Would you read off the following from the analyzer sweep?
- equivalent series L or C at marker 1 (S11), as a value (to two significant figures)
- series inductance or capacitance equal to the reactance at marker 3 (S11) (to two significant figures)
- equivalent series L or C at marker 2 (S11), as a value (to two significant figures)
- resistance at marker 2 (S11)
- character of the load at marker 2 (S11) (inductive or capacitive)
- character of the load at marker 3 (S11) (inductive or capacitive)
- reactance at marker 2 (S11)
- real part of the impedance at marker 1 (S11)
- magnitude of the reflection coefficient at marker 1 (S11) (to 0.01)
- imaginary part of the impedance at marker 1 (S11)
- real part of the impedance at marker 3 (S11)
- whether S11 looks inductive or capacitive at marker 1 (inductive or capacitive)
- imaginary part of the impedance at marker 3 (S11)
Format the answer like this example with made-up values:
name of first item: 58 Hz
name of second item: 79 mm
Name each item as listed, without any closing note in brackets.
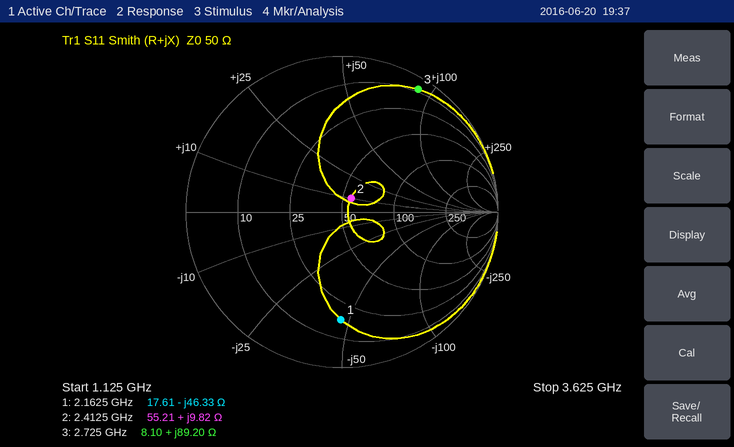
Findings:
equivalent series L or C at marker 1 (S11), as a value: 1.6 pF
series inductance or capacitance equal to the reactance at marker 3 (S11): 5.2 nH
equivalent series L or C at marker 2 (S11), as a value: 650 pH
resistance at marker 2: 55.21 Ω
character of the load at marker 2 (S11): inductive
character of the load at marker 3 (S11): inductive
reactance at marker 2: +9.82 Ω
real part of the impedance at marker 1: 17.61 Ω
magnitude of the reflection coefficient at marker 1 (S11): 0.69
imaginary part of the impedance at marker 1: -46.33 Ω
real part of the impedance at marker 3: 8.10 Ω
whether S11 looks inductive or capacitive at marker 1: capacitive
imaginary part of the impedance at marker 3: +89.20 Ω
